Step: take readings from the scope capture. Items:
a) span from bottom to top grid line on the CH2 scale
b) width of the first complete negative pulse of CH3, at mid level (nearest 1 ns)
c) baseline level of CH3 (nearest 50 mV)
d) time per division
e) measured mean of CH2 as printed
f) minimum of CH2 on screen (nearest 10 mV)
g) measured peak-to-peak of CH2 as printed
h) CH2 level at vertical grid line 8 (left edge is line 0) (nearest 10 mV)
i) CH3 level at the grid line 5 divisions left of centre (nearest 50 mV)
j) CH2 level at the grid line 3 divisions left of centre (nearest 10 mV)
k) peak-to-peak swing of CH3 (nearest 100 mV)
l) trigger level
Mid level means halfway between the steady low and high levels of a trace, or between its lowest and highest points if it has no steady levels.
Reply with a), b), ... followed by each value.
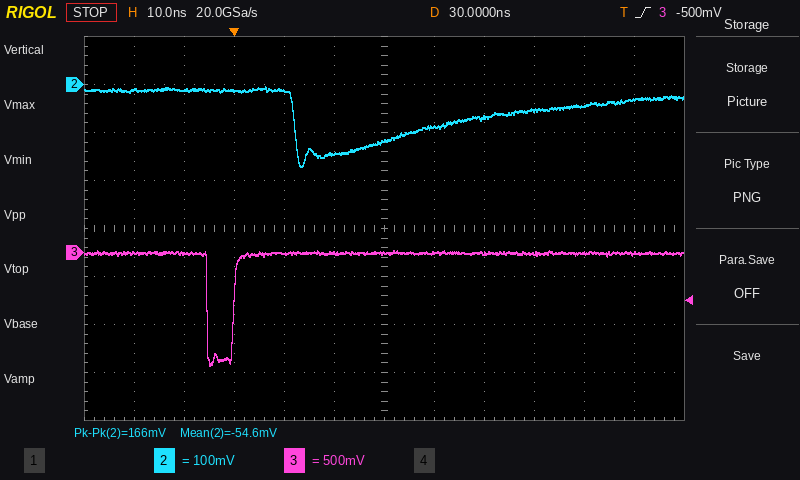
a) 800 mV
b) 5 ns
c) 0 mV
d) 10 ns
e) -54.6 mV
f) -170 mV
g) 166 mV
h) -70 mV
i) 0 mV
j) -10 mV
k) 1.20 V
l) -500 mV
